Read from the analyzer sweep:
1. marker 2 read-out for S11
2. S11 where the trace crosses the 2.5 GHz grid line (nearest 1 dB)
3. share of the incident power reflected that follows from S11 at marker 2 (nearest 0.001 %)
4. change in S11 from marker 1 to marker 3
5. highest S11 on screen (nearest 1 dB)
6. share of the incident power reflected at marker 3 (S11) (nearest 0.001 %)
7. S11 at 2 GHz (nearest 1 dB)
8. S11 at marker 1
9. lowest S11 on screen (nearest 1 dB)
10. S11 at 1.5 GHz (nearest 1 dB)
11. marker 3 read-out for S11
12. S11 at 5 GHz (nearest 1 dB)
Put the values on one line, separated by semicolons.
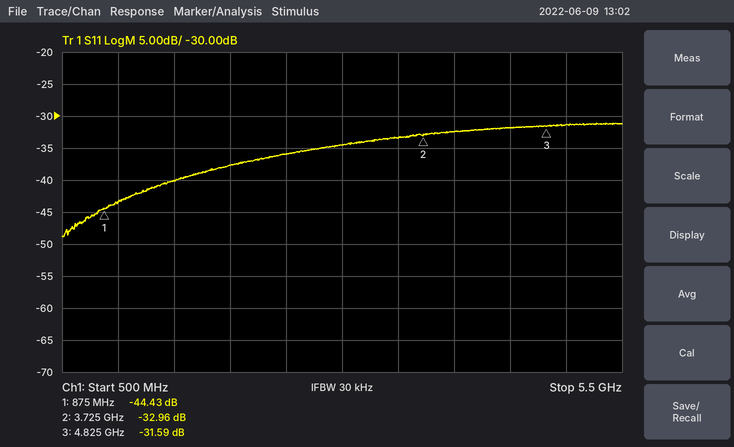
-32.96 dB; -36 dB; 0.051 %; 12.84 dB; -31 dB; 0.069 %; -38 dB; -44.43 dB; -49 dB; -40 dB; -31.59 dB; -31 dB
